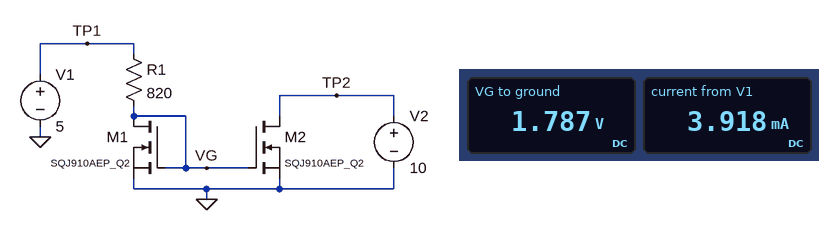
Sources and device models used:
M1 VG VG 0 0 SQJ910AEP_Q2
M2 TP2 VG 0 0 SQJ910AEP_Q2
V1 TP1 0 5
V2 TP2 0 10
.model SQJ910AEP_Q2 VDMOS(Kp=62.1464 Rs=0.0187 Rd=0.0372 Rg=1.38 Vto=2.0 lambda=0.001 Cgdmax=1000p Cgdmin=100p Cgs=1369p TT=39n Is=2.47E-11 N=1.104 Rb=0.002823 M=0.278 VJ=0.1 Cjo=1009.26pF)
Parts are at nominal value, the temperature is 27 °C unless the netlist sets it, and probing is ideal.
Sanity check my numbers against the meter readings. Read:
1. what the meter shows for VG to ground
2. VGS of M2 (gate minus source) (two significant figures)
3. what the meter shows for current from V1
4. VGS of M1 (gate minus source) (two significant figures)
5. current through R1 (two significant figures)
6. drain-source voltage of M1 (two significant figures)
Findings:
1.787 V
1.8 V
3.918 mA
1.8 V
3.9 mA
1.8 V
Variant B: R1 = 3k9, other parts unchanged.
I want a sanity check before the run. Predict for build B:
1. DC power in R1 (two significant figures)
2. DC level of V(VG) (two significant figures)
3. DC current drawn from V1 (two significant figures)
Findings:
2.8 mW
1.7 V
840 µA
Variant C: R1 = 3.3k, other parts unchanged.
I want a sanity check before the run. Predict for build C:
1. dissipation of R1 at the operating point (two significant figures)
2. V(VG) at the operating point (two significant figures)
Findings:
3.3 mW
1.7 V
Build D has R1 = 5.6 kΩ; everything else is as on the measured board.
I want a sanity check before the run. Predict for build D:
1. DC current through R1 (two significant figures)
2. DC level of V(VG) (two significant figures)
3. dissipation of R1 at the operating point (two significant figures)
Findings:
590 µA
1.7 V
2.0 mW
